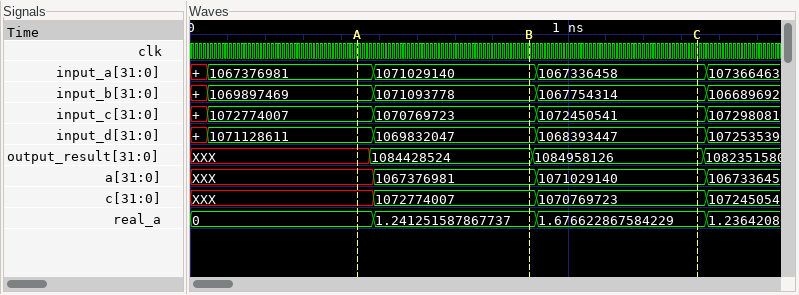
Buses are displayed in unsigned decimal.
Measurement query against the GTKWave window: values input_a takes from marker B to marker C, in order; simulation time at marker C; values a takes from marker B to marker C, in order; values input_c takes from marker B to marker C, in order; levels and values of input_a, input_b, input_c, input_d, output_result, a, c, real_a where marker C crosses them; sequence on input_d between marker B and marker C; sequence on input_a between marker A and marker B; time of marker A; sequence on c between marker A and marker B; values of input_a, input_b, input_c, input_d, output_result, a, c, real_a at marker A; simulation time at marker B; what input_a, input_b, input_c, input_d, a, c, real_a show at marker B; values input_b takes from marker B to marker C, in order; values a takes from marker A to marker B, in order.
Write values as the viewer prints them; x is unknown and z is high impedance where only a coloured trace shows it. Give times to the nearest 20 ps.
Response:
1071029140, 1067336458
1340 ps
1067376981, 1071029140
1070769723, 1072450541
input_a=1067336458, input_b=1067754314, input_c=1072450541, input_d=1068393447, output_result=1084958126, a=1071029140, c=1070769723, real_a=1.676622867584229
1069832047, 1068393447
1067376981, 1071029140
440 ps
XXX, 1072774007
input_a=1067376981, input_b=1069897469, input_c=1072774007, input_d=1071128611, output_result=XXX, a=XXX, c=XXX, real_a=0
900 ps
input_a=1071029140, input_b=1071093778, input_c=1070769723, input_d=1069832047, a=1067376981, c=1072774007, real_a=1.241251587867737
1071093778, 1067754314
XXX, 1067376981
